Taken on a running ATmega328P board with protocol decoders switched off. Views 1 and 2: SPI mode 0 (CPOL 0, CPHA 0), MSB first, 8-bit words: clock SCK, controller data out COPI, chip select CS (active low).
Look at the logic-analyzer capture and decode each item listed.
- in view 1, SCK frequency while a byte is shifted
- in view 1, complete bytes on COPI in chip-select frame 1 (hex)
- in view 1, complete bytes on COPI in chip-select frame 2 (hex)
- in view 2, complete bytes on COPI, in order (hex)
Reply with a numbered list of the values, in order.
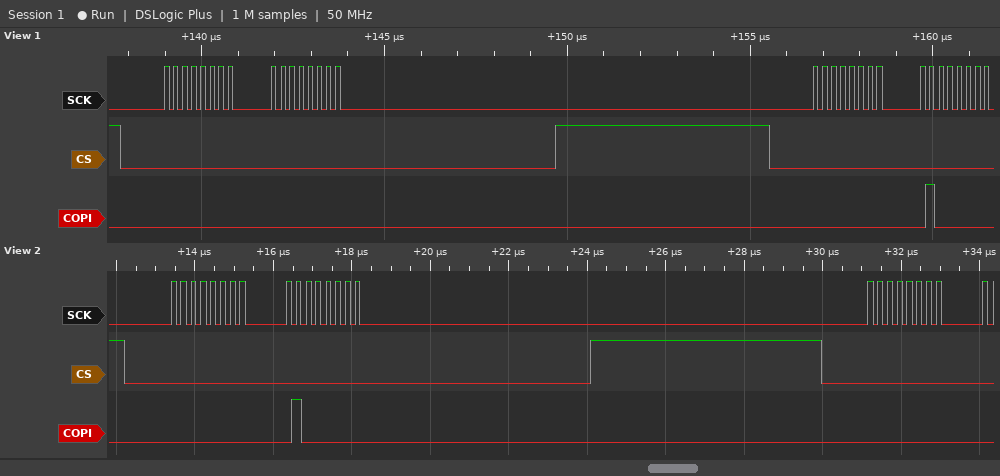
1. 4 MHz
2. 00 00
3. 00 40
4. 00 40 00
